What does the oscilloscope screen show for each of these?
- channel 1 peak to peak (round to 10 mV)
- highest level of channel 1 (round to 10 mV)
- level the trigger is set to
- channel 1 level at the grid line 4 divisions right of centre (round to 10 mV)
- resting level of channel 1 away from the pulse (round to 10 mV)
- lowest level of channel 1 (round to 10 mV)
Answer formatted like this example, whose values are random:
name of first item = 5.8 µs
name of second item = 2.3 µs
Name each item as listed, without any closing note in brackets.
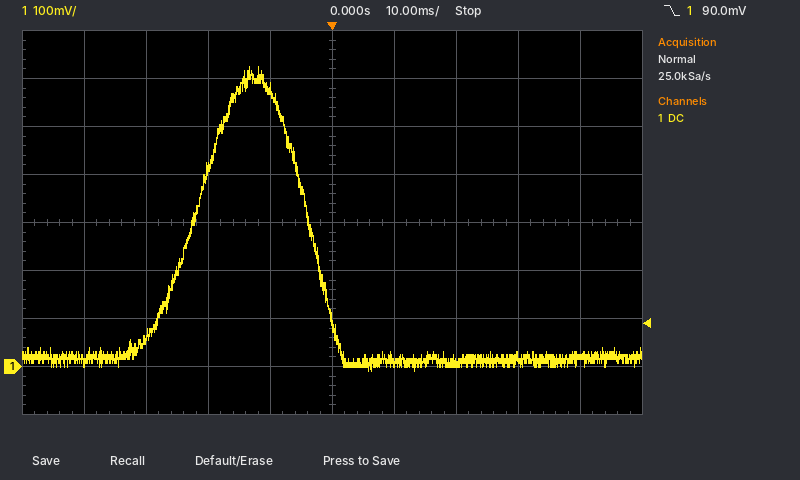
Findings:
channel 1 peak to peak = 630 mV
highest level of channel 1 = 620 mV
level the trigger is set to = 90.0 mV
channel 1 level at the grid line 4 divisions right of centre = 20 mV
resting level of channel 1 away from the pulse = 20 mV
lowest level of channel 1 = -10 mV
